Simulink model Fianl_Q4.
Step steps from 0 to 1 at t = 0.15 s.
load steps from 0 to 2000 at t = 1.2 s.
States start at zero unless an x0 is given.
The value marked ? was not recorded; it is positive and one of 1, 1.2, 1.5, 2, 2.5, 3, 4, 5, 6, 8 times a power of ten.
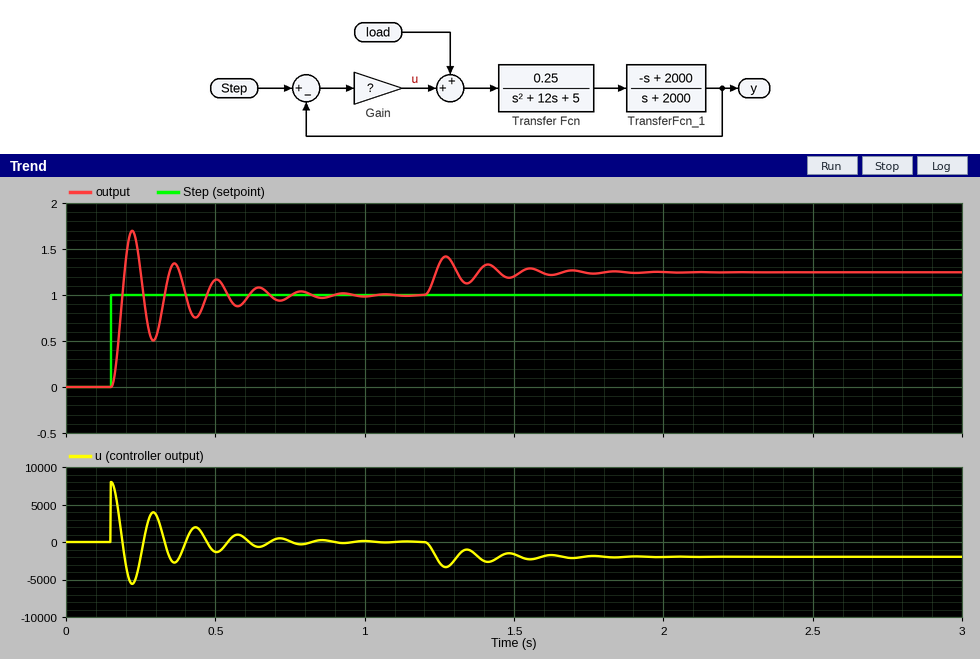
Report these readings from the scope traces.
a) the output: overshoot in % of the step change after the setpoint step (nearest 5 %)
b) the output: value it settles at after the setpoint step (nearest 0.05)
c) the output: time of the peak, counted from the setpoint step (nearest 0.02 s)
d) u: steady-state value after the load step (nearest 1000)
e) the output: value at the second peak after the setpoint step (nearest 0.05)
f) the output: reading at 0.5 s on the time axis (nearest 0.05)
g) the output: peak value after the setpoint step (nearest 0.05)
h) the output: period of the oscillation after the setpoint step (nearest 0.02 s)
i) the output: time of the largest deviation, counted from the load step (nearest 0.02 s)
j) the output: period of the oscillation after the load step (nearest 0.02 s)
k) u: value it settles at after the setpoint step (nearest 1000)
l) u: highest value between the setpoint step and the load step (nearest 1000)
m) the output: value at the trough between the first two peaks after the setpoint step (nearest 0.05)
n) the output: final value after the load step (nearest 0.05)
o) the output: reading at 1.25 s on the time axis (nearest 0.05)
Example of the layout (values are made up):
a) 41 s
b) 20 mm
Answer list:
a) 70 %
b) 1.00
c) 0.08 s
d) -2000
e) 1.35
f) 1.15
g) 1.70
h) 0.14 s
i) 0.08 s
j) 0.14 s
k) 0
l) 8000
m) 0.50
n) 1.25
o) 1.35
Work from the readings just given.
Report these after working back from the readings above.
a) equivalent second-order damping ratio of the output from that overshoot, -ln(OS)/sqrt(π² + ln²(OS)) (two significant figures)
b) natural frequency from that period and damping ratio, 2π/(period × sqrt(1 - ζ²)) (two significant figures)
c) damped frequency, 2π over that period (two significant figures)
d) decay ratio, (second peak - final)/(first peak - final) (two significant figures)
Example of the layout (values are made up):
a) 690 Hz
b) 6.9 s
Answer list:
a) 0.11
b) 45 rad/s
c) 45 rad/s
d) 0.50
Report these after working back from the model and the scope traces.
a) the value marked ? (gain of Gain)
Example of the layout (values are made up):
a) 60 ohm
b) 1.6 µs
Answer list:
a) 8000
